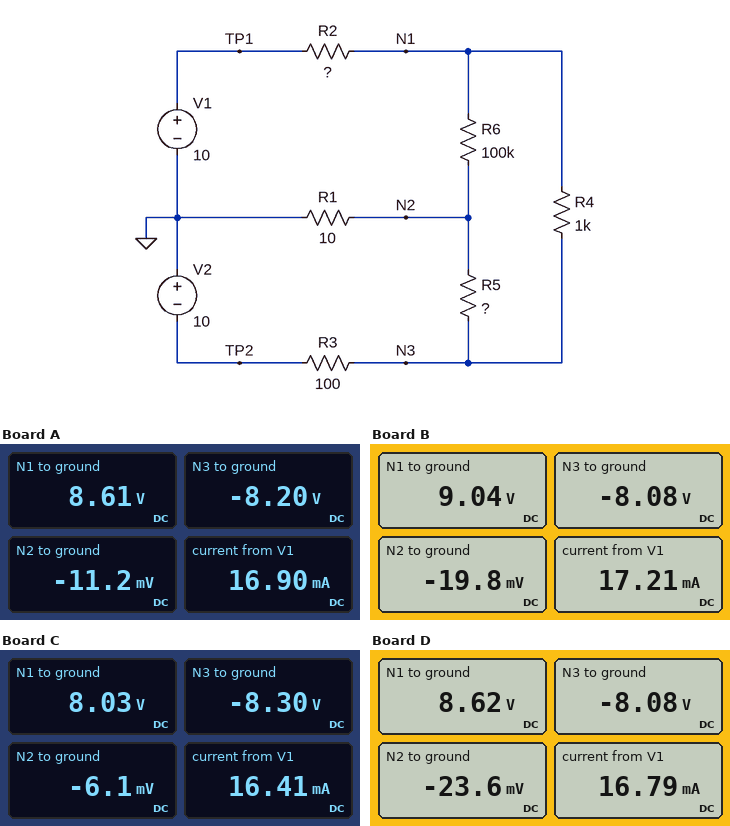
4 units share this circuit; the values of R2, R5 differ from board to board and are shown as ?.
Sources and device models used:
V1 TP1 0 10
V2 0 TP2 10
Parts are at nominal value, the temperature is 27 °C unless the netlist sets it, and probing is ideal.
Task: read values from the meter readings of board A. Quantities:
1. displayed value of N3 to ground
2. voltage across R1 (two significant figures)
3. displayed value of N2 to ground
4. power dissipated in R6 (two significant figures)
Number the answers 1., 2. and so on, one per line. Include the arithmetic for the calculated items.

1. -8.20 V
2. 0 V - (-11.2 mV) = 11 mV
3. -11.2 mV
4. (8.61 V - (-11.2 mV))^2 / 100 kΩ = 740 µW
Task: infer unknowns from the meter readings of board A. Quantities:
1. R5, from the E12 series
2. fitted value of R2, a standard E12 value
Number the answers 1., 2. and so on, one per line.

1. 6.8 kΩ
2. 82 Ω
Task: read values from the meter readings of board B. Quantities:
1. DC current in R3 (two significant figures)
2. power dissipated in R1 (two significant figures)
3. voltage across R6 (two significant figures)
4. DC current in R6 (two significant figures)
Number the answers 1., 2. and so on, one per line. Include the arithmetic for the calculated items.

1. (-8.08 V - (-10 V)) / 100 Ω = 19 mA
2. (0 V - (-19.8 mV))^2 / 10 Ω = 39 µW
3. 9.04 V - (-19.8 mV) = 9.1 V
4. (9.04 V - (-19.8 mV)) / 100 kΩ = 91 µA
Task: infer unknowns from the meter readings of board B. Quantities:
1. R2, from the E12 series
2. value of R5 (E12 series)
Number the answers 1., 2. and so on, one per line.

1. 56 Ω
2. 3.9 kΩ
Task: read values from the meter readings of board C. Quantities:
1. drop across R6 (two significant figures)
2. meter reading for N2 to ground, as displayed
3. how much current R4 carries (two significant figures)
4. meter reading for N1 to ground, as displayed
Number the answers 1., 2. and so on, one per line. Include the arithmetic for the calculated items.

1. 8.03 V - (-6.1 mV) = 8.0 V
2. -6.1 mV
3. (8.03 V - (-8.3 V)) / 1 kΩ = 16 mA
4. 8.03 V
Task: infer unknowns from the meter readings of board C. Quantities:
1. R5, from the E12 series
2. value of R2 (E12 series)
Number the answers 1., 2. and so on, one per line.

1. 12 kΩ
2. 120 Ω
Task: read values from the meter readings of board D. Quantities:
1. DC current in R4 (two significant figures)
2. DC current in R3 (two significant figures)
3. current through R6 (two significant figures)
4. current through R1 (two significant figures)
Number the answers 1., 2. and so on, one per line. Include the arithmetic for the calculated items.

1. (8.62 V - (-8.08 V)) / 1 kΩ = 17 mA
2. (-8.08 V - (-10 V)) / 100 Ω = 19 mA
3. (8.62 V - (-23.6 mV)) / 100 kΩ = 86 µA
4. (0 V - (-23.6 mV)) / 10 Ω = 2.4 mA
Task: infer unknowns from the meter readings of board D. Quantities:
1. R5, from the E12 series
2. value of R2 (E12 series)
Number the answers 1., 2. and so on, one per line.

1. 3.3 kΩ
2. 82 Ω
